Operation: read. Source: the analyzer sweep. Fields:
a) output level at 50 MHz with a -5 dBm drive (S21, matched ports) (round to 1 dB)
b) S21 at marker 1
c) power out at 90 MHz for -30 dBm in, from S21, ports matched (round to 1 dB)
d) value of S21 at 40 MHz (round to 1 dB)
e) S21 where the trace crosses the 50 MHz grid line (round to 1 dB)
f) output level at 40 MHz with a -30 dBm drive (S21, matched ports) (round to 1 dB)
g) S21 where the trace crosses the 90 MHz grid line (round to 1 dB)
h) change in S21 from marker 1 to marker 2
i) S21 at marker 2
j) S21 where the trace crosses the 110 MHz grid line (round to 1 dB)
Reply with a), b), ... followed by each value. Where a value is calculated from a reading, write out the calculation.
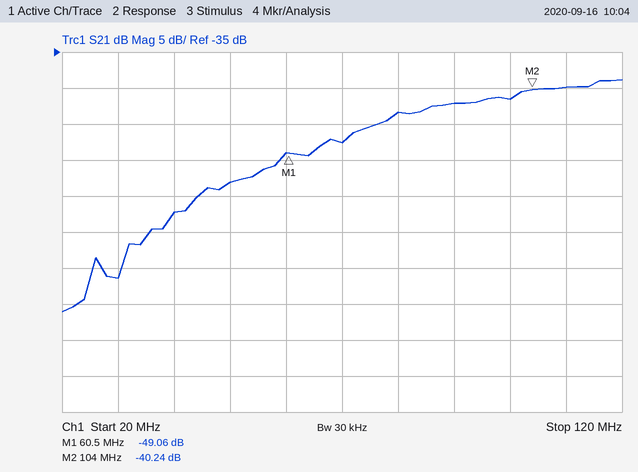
a) -5 dBm + (-53 dB) = -58 dBm
b) -49.06 dB
c) -30 dBm + (-42 dB) = -72 dBm
d) -57 dB
e) -53 dB
f) -30 dBm + (-57 dB) = -87 dBm
g) -42 dB
h) -40.24 − (-49.06) = 8.82 dB
i) -40.24 dB
j) -40 dB
